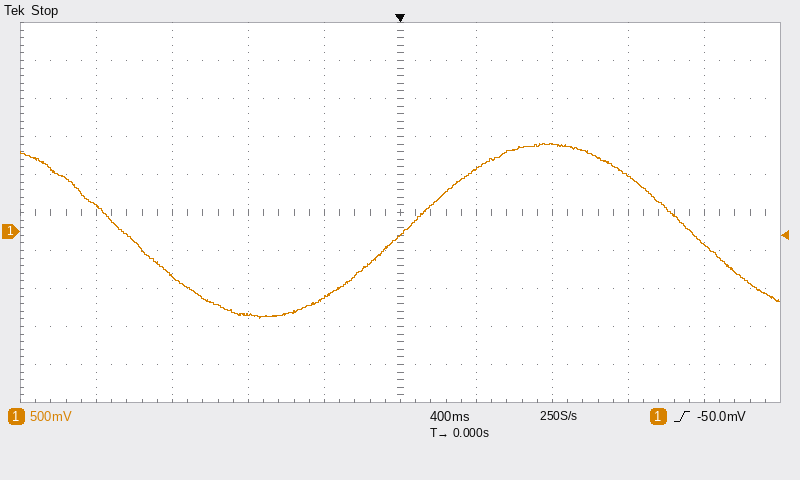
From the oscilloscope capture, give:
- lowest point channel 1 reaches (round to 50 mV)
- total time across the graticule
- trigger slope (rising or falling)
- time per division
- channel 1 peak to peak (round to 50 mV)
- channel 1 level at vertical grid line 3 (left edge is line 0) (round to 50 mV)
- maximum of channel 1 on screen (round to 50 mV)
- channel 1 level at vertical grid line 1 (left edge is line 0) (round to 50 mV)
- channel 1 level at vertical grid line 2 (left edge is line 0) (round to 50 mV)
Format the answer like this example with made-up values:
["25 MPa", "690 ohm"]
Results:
["-1.15 V", "4 s", "rising", "400 ms", "2.30 V", "-1.10 V", "1.15 V", "350 mV", "-600 mV"]
